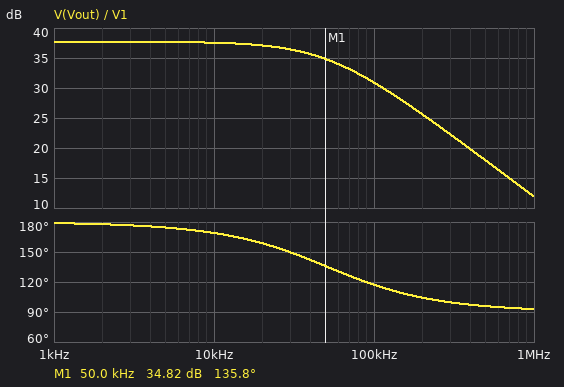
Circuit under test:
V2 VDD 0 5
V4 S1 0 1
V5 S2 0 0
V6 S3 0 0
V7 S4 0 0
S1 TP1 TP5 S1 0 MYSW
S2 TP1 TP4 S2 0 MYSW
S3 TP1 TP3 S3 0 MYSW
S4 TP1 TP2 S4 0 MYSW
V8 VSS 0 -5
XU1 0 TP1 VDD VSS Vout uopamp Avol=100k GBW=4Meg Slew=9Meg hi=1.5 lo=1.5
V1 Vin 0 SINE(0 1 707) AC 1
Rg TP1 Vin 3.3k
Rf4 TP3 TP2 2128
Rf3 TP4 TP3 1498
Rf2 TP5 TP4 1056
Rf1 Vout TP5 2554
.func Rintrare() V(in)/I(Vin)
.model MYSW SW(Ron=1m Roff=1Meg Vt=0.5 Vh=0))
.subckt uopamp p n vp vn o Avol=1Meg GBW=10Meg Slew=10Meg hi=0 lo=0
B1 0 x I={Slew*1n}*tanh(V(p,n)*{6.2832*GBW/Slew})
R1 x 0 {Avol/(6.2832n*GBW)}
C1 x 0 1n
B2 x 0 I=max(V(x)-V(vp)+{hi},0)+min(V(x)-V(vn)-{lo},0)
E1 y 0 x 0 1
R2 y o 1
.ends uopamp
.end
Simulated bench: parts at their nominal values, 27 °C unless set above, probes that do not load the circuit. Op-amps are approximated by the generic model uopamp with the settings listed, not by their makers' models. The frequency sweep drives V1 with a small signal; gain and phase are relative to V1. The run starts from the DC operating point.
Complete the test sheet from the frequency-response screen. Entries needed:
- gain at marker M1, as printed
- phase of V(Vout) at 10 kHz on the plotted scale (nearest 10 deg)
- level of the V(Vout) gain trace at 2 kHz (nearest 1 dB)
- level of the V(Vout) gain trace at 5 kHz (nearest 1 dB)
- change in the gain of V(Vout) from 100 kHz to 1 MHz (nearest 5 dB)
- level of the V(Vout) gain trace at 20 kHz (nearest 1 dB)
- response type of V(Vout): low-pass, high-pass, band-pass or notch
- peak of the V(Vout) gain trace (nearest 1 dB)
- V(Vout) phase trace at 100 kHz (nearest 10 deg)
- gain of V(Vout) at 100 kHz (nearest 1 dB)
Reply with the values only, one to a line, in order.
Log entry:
34.82 dB
170 deg
38 dB
38 dB
-20 dB
37 dB
low-pass
38 dB
120 deg
31 dB
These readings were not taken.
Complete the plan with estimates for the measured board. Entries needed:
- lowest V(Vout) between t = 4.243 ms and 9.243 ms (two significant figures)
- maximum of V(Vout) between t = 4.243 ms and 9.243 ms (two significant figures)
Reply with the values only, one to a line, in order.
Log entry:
-770 mV
770 mV
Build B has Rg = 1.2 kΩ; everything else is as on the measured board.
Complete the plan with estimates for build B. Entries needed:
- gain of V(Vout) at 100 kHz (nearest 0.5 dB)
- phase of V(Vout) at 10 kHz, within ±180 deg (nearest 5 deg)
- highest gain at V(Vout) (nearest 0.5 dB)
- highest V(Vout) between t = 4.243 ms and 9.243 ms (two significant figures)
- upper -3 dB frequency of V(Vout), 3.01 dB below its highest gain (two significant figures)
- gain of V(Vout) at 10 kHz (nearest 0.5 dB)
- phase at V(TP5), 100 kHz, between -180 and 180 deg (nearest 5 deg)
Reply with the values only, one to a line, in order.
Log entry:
32.0 dB
150 deg
46.5 dB
2.1 V
19 kHz
45.5 dB
100 deg
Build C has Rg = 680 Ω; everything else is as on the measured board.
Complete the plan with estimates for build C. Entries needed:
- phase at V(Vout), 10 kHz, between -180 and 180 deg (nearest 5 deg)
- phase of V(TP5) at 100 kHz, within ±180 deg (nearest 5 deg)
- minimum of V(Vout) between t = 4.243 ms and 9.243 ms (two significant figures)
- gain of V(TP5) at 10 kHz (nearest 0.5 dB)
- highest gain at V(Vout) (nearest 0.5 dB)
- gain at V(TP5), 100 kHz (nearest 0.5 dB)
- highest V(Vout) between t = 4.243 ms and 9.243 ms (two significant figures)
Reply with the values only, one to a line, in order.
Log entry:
135 deg
95 deg
-3.5 V
48.5 dB
51.5 dB
32.0 dB
3.5 V
